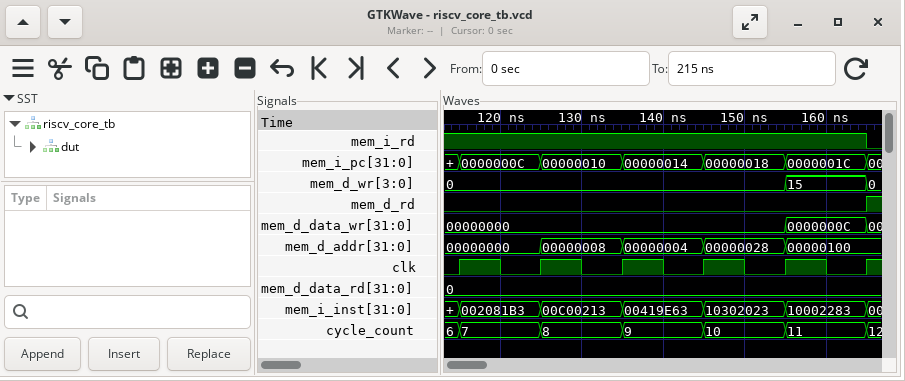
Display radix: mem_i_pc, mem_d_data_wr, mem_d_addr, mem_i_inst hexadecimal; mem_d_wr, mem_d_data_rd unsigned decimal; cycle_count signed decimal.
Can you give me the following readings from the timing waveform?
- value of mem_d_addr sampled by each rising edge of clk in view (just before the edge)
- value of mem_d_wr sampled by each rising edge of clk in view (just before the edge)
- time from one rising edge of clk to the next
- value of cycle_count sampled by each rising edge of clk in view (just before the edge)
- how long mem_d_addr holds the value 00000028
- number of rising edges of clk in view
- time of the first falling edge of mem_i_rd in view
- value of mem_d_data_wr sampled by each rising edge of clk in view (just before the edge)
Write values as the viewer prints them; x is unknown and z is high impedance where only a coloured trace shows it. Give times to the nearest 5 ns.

00000000, 00000000, 00000008, 00000004, 00000028, 00000100
0, 0, 0, 0, 0, 15
10 ns
6, 7, 8, 9, 10, 11
10 ns
6
165 ns
00000000, 00000000, 00000000, 00000000, 00000000, 0000000C
